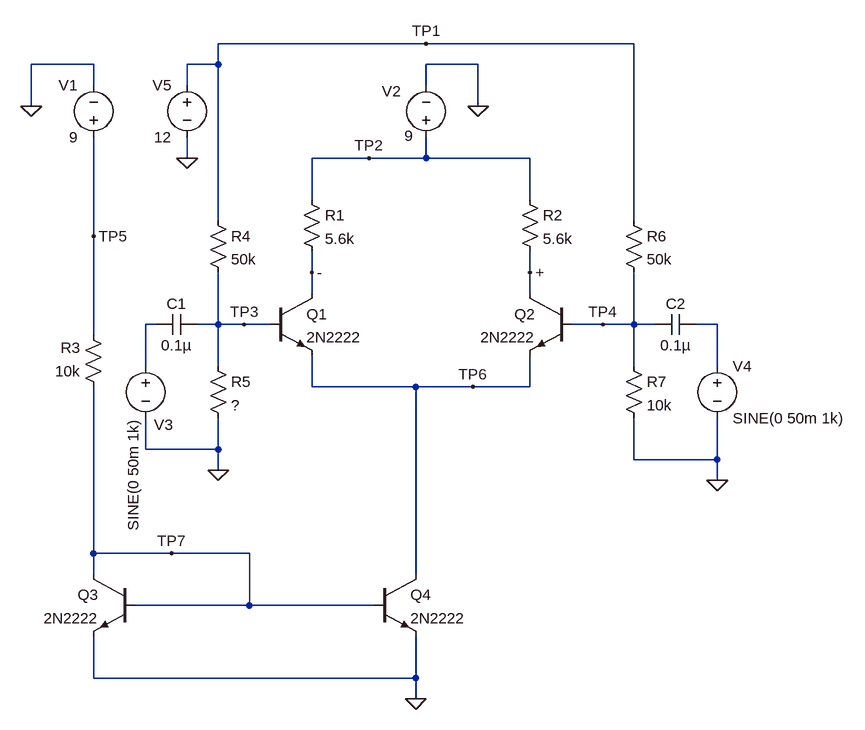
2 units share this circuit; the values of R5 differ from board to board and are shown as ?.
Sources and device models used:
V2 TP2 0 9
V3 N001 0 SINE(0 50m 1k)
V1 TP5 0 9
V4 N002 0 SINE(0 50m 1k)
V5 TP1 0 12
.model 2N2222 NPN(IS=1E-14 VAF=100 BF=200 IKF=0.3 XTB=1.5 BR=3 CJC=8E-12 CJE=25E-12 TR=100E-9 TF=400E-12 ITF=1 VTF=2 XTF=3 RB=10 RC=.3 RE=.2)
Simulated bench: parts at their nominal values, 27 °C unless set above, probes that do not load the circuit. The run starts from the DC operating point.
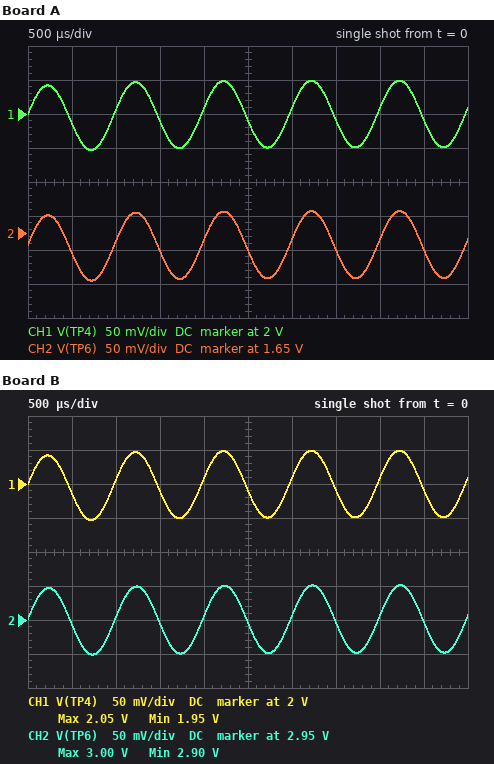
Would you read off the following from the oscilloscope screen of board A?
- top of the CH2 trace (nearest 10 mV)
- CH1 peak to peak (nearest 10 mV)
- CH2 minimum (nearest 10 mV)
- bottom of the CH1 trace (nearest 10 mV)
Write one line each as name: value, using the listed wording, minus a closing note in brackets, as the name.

top of the CH2 trace: 1.68 V
CH1 peak to peak: 100 mV
CH2 minimum: 1.58 V
bottom of the CH1 trace: 1.95 V
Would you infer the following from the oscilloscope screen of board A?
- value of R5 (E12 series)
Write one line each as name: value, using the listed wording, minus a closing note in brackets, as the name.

value of R5: 12 kΩ
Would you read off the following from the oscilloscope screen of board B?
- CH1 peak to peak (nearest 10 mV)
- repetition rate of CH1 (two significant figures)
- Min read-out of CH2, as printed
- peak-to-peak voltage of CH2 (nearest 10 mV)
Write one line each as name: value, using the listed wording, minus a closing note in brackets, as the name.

CH1 peak to peak: 100 mV
repetition rate of CH1: 1.0 kHz
Min read-out of CH2, as printed: 2.90 V
peak-to-peak voltage of CH2: 100 mV
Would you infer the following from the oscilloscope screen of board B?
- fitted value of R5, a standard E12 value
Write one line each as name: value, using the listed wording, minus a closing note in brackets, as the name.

fitted value of R5, a standard E12 value: 22 kΩ
